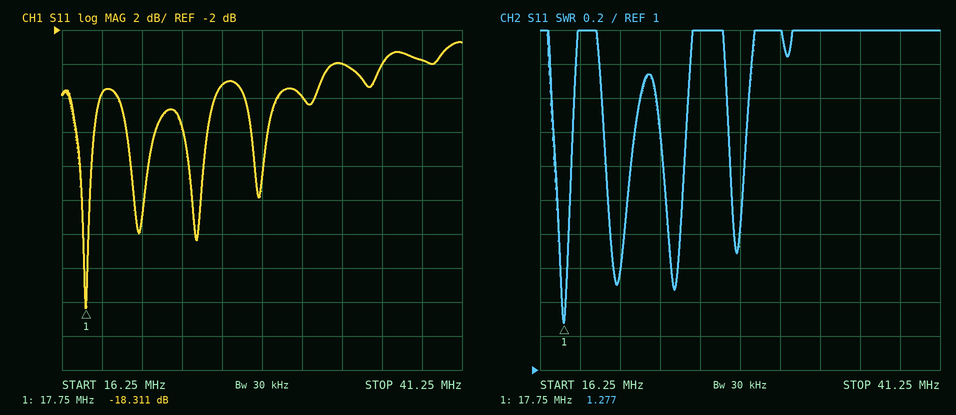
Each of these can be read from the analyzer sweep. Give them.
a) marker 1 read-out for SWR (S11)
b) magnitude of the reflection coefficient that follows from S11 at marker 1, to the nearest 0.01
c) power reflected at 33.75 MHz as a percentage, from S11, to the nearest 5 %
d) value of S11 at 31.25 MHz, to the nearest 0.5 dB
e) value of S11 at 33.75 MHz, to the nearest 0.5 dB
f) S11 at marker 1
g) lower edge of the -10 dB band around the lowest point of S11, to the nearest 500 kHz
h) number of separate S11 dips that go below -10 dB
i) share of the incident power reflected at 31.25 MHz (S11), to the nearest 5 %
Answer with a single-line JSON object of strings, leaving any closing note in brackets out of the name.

{"marker 1 read-out for SWR": "1.277", "magnitude of the reflection coefficient that follows from S11 at marker 1, to the nearest 0.01": "0.12", "power reflected at 33.75 MHz as a percentage, from S11, to the nearest 5 %": "40 %", "value of S11 at 31.25 MHz, to the nearest 0.5 dB": "-6.0 dB", "value of S11 at 33.75 MHz, to the nearest 0.5 dB": "-4.0 dB", "S11 at marker 1": "-18.311 dB", "lower edge of the -10 dB band around the lowest point of S11, to the nearest 500 kHz": "17.5 MHz", "number of separate S11 dips that go below -10 dB": "4", "share of the incident power reflected at 31.25 MHz (S11), to the nearest 5 %": "25 %"}
